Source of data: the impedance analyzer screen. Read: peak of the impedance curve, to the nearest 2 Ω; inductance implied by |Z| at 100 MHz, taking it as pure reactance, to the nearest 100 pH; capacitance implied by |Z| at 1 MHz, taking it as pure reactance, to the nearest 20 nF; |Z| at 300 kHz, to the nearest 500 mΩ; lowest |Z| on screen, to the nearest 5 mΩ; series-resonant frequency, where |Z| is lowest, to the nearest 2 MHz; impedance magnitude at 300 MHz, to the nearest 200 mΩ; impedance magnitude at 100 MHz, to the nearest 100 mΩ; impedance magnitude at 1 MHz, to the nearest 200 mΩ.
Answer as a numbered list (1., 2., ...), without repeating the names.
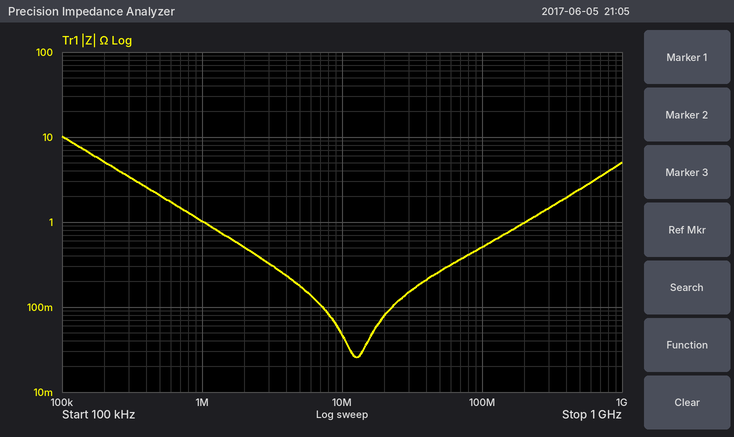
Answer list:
1. 10 Ω
2. 800 pH
3. 160 nF
4. 3.5 Ω
5. 25 mΩ
6. 12 MHz
7. 1.4 Ω
8. 500 mΩ
9. 1.0 Ω
